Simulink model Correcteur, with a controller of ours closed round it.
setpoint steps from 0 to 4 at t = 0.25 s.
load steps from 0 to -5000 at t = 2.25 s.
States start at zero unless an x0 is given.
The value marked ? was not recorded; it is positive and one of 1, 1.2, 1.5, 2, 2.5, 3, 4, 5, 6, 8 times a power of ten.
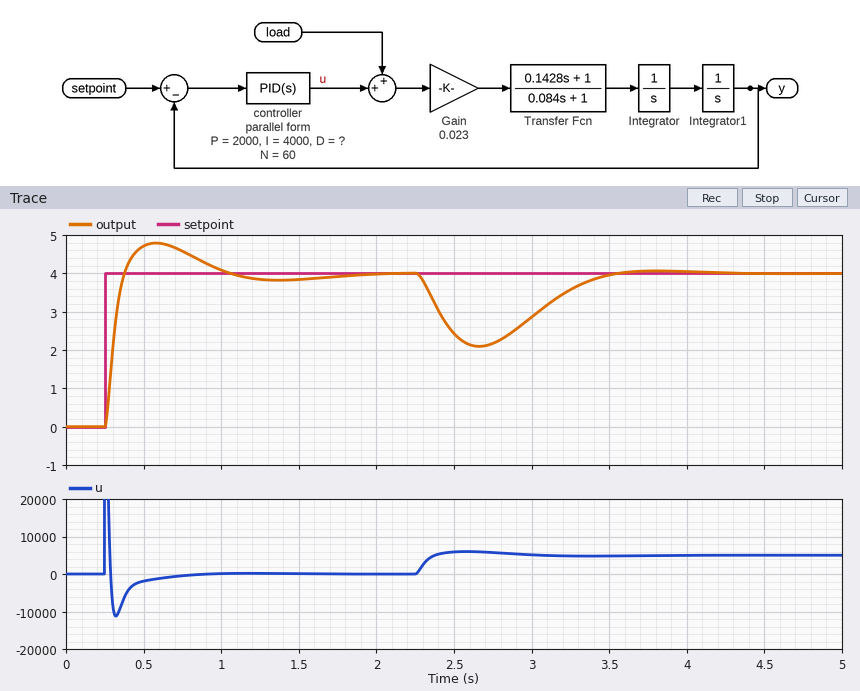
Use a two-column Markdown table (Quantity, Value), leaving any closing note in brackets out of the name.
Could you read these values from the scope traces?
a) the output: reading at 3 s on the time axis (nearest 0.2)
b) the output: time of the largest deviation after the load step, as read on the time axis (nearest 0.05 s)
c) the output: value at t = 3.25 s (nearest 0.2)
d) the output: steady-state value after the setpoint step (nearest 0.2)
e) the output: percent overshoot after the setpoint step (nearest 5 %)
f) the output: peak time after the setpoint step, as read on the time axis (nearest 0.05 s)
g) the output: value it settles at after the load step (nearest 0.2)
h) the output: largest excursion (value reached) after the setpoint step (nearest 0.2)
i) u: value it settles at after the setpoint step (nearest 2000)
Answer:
| Quantity | Value |
|---|---|
| the output: reading at 3 s on the time axis | 2.8 |
| the output: time of the largest deviation after the load step, as read on the time axis | 2.65 s |
| the output: value at t = 3.25 s | 3.6 |
| the output: steady-state value after the setpoint step | 4.0 |
| the output: percent overshoot after the setpoint step | 20 % |
| the output: peak time after the setpoint step, as read on the time axis | 0.60 s |
| the output: value it settles at after the load step | 4.0 |
| the output: largest excursion (value reached) after the setpoint step | 4.8 |
| u: value it settles at after the setpoint step | 0 |
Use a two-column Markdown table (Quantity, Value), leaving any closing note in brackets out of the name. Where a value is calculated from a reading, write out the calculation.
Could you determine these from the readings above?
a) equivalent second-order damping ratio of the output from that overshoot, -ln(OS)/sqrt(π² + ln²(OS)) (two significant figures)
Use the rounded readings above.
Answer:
| Quantity | Value |
|---|---|
| equivalent second-order damping ratio of the output from that overshoot, -ln(OS)/sqrt(π² + ln²(OS)) | ln(0.2) = -1.609; 1.609 / sqrt(9.870 + 2.590) = 0.46 |
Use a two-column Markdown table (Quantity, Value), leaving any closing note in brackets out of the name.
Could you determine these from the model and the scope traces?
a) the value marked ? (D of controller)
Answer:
| Quantity | Value |
|---|---|
| the value marked ? | 400 |
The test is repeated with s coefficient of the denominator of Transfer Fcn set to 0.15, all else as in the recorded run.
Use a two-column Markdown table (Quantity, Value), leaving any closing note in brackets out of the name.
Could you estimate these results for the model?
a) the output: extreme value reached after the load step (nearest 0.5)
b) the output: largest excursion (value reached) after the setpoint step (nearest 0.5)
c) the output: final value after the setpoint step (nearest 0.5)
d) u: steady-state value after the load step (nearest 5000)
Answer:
| Quantity | Value |
|---|---|
| the output: extreme value reached after the load step | 2.0 |
| the output: largest excursion (value reached) after the setpoint step | 5.5 |
| the output: final value after the setpoint step | 4.0 |
| u: steady-state value after the load step | 5000 |
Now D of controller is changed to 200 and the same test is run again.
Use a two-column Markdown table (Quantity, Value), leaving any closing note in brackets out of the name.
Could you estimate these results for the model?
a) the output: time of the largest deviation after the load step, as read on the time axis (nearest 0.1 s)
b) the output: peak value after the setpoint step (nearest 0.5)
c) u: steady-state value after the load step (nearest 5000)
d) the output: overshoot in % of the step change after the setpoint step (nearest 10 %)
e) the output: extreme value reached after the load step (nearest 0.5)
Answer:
| Quantity | Value |
|---|---|
| the output: time of the largest deviation after the load step, as read on the time axis | 2.6 s |
| the output: peak value after the setpoint step | 5.5 |
| u: steady-state value after the load step | 5000 |
| the output: overshoot in % of the step change after the setpoint step | 40 % |
| the output: extreme value reached after the load step | 1.5 |
